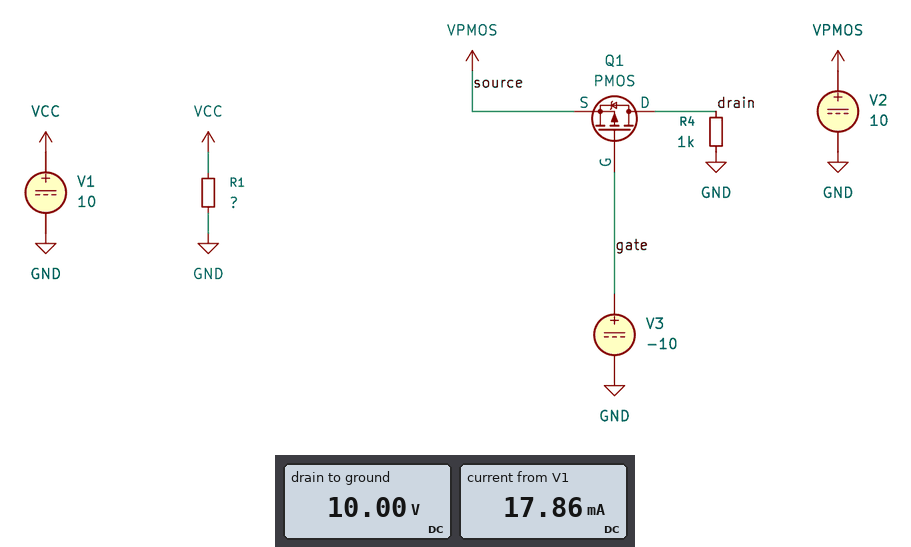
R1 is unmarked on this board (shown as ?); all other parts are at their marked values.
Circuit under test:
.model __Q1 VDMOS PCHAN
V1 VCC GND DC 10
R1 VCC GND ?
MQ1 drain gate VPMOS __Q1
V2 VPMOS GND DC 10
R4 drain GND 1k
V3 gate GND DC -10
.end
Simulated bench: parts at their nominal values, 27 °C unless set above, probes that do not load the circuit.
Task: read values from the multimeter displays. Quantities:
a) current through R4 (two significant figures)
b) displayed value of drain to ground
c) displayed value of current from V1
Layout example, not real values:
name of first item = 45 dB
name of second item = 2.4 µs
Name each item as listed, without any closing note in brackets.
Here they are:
current through R4 = 10 mA
displayed value of drain to ground = 10.00 V
displayed value of current from V1 = 17.86 mA
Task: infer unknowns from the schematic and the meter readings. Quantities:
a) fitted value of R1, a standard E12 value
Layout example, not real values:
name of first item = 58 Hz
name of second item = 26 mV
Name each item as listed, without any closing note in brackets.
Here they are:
fitted value of R1, a standard E12 value = 560 Ω
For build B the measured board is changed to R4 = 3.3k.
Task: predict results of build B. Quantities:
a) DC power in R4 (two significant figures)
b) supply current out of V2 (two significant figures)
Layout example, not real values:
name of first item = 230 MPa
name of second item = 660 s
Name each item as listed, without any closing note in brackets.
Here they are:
DC power in R4 = 30 mW
supply current out of V2 = 3.0 mA
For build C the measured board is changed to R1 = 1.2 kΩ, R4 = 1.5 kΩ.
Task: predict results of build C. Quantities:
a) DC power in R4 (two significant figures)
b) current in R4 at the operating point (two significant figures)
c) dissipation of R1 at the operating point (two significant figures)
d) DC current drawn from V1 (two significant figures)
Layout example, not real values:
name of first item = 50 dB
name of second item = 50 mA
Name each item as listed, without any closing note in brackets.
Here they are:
DC power in R4 = 67 mW
current in R4 at the operating point = 6.7 mA
dissipation of R1 at the operating point = 83 mW
DC current drawn from V1 = 8.3 mA
